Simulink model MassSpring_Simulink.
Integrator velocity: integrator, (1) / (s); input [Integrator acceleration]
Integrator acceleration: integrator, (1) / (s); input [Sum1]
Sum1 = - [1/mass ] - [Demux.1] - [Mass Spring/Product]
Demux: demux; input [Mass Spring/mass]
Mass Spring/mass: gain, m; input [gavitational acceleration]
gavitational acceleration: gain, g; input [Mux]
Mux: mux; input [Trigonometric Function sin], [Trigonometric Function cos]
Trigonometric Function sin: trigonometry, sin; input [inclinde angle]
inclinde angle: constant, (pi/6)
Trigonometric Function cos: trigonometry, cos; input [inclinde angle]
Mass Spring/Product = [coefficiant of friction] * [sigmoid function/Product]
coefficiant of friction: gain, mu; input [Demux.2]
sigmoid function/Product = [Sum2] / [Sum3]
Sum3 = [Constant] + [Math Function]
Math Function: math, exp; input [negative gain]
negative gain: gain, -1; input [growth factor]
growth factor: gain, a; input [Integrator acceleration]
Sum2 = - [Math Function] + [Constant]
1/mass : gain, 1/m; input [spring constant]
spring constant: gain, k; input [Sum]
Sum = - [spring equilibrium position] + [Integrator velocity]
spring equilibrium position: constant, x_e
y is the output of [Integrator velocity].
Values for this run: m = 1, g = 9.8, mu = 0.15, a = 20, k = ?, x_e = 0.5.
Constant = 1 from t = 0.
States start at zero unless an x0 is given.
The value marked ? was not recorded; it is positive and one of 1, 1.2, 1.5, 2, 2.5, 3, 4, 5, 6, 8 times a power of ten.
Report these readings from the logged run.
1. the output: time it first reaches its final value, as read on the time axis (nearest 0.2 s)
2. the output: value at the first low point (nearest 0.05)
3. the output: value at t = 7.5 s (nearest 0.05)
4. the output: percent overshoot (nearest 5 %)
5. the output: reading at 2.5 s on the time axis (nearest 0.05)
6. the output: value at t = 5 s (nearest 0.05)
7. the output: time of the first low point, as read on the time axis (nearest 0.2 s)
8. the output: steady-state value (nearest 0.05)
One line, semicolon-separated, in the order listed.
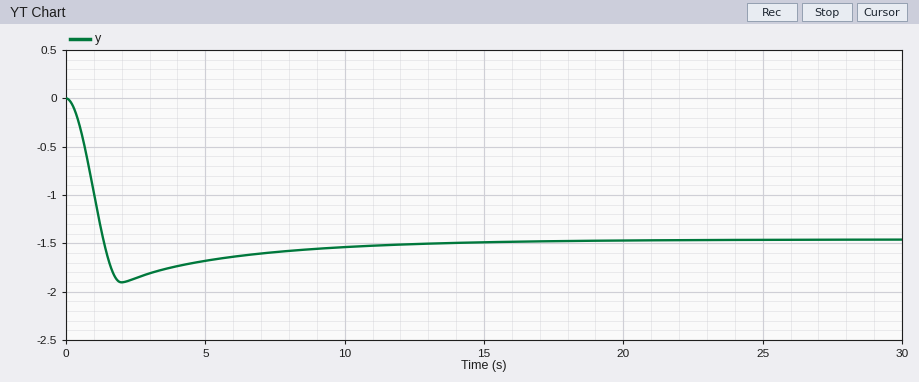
1.4 s; -1.90; -1.60; 30 %; -1.85; -1.70; 2.0 s; -1.45
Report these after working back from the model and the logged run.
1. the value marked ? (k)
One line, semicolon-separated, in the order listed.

2.5
